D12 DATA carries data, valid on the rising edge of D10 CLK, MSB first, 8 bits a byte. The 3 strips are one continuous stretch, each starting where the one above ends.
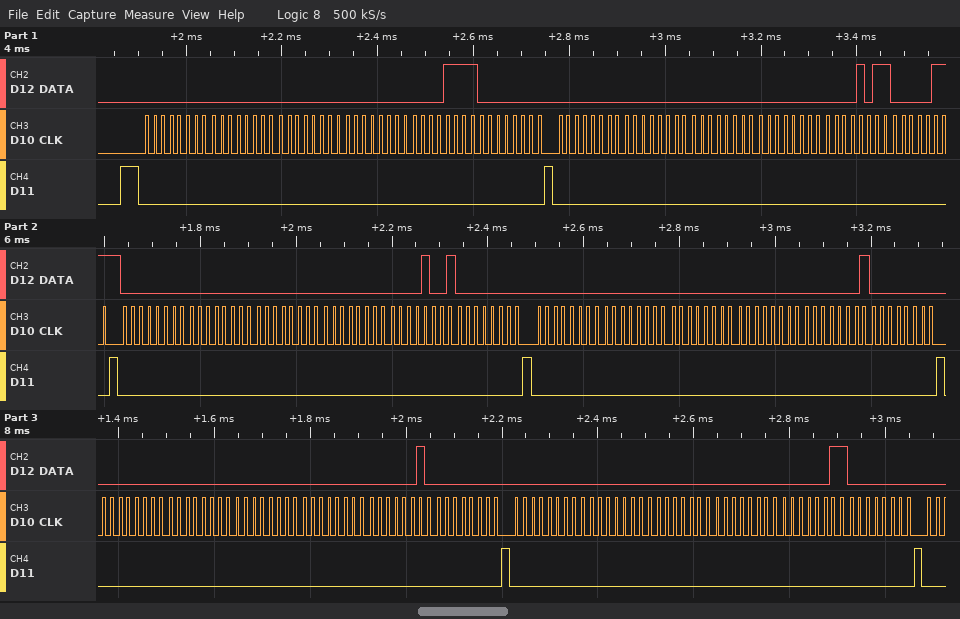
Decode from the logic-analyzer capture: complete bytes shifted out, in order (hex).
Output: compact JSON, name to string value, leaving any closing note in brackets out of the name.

{"complete bytes shifted out, in order": "00 00 00 00 0F 00 00 00 00 00 0B 07 00 00 00 00 09 00 00 00 00 00 01 00 00 00 00 00 02 00 00 00 00 00 03 00"}
